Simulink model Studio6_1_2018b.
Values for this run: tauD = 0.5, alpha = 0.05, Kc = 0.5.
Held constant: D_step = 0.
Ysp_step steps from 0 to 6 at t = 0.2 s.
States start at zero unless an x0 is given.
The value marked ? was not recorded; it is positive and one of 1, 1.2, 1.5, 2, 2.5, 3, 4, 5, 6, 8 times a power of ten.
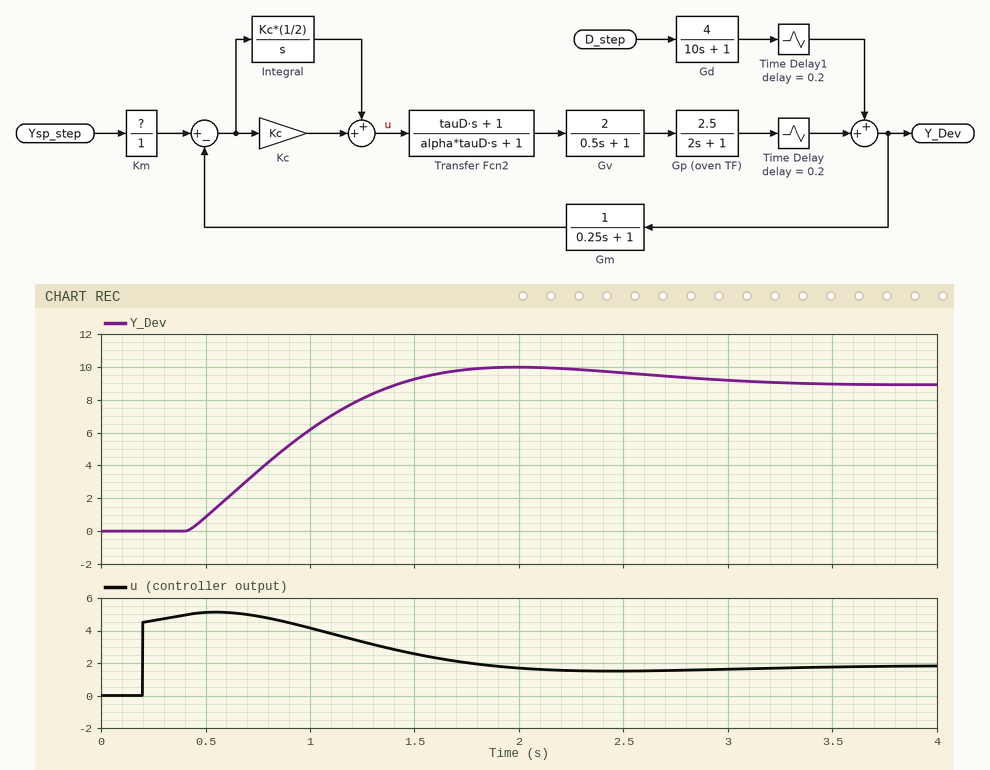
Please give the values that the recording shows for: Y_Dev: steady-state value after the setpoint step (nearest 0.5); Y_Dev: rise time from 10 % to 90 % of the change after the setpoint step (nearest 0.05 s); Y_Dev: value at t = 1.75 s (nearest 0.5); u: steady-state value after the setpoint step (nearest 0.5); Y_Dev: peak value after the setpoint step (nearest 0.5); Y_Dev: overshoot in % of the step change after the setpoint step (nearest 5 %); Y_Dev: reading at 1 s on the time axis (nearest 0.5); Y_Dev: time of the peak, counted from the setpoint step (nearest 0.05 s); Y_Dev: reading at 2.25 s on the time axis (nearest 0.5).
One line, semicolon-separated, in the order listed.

9.0; 0.75 s; 10.0; 2.0; 10.0; 10 %; 6.0; 1.80 s; 10.0
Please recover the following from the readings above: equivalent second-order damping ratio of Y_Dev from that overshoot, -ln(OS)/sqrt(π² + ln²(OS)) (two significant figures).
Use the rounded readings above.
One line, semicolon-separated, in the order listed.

0.59
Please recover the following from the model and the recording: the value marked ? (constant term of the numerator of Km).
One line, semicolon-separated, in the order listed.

1.5
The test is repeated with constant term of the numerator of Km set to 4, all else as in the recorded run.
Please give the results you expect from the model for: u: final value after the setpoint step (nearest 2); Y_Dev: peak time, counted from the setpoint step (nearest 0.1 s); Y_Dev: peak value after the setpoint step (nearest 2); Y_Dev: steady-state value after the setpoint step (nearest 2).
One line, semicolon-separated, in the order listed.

4; 1.8 s; 26; 24
